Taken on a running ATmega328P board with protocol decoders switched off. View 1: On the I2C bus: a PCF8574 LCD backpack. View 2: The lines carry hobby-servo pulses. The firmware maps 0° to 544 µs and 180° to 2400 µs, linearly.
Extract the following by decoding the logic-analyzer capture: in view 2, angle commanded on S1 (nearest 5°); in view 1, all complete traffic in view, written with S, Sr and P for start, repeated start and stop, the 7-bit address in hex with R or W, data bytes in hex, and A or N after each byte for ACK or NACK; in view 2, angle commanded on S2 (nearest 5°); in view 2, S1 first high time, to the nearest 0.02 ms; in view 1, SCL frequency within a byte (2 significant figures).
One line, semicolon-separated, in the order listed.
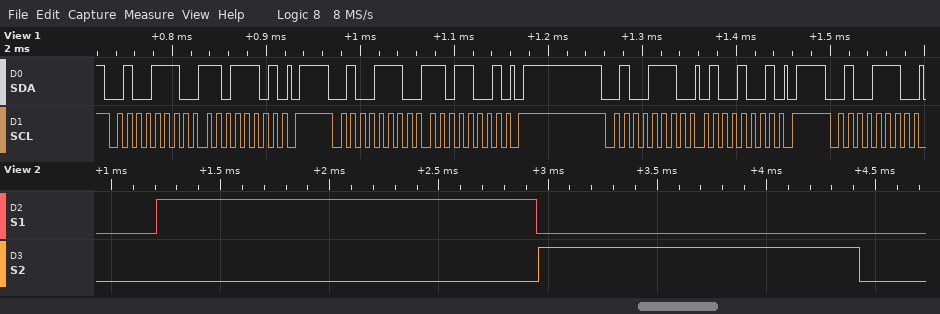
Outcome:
115°; S 27W A DD A P S 27W A D9 A P S 27W A 49 A P S 27W A; 90°; 1.74 ms; 100 kHz
